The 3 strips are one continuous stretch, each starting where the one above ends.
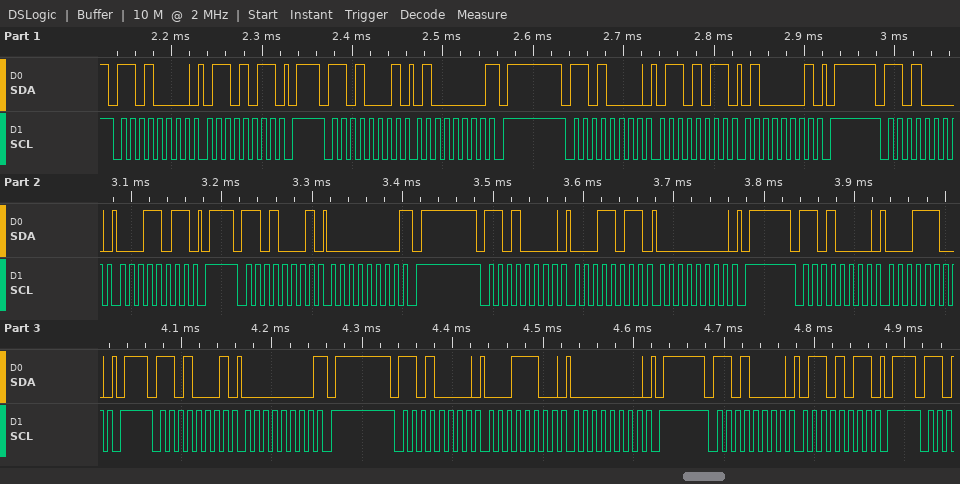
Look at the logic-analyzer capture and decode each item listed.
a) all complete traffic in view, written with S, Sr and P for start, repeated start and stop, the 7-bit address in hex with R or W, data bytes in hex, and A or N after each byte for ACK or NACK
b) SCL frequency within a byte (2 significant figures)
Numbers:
S 68W A 6B A P S 68R A 40 N P S 68W A 6B A 41 A P S 68W A 1B A P S 68R A 00 N P S 68W A 1B A 00 A P S 68W A 1C A P S 68R A 00 N P S 68W A 1C A 00 A P S 68W A 6B A P
100 kHz
